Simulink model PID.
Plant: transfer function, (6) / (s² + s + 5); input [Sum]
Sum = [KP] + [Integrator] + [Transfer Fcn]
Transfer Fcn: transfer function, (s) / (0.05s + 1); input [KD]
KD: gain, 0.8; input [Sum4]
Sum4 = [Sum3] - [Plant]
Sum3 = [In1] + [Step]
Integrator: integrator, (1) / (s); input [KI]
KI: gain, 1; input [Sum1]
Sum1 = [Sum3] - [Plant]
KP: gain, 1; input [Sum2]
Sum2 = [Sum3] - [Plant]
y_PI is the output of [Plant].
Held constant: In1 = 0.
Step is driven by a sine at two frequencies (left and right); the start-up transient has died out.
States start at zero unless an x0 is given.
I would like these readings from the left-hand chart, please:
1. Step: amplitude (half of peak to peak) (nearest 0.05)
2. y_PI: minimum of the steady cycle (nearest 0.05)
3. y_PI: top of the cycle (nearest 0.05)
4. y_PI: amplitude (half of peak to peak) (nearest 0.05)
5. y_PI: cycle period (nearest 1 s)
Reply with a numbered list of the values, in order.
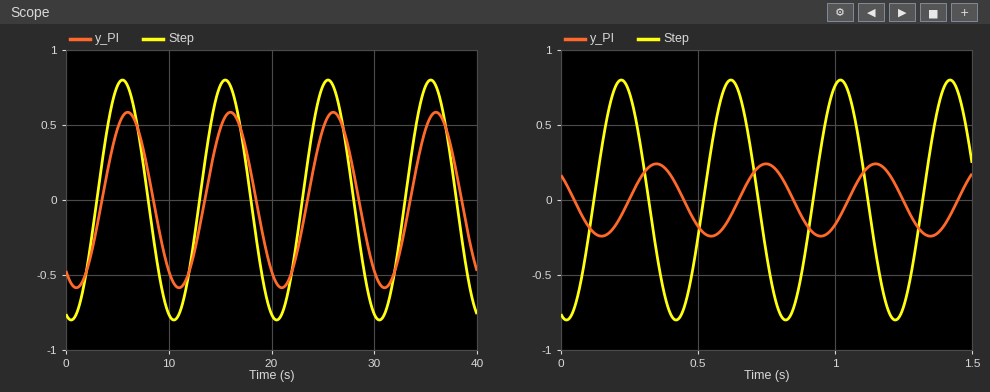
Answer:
1. 0.80
2. -0.60
3. 0.60
4. 0.60
5. 10 s
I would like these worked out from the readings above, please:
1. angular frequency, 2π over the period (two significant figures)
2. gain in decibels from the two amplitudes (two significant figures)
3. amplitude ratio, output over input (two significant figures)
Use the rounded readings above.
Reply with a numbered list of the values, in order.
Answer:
1. 0.63 rad/s
2. -2.5 dB
3. 0.75
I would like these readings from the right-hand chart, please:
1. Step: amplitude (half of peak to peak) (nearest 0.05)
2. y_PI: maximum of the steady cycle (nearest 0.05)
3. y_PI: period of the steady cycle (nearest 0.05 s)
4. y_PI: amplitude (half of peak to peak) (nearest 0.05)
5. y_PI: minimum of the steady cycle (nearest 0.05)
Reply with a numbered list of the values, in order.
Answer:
1. 0.80
2. 0.25
3. 0.40 s
4. 0.25
5. -0.25
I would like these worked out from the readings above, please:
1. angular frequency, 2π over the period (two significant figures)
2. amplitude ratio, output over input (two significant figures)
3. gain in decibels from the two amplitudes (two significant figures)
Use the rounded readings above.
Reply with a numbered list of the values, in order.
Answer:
1. 16 rad/s
2. 0.31
3. -10 dB
